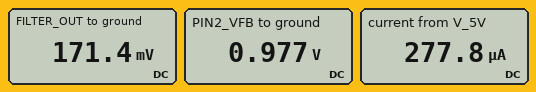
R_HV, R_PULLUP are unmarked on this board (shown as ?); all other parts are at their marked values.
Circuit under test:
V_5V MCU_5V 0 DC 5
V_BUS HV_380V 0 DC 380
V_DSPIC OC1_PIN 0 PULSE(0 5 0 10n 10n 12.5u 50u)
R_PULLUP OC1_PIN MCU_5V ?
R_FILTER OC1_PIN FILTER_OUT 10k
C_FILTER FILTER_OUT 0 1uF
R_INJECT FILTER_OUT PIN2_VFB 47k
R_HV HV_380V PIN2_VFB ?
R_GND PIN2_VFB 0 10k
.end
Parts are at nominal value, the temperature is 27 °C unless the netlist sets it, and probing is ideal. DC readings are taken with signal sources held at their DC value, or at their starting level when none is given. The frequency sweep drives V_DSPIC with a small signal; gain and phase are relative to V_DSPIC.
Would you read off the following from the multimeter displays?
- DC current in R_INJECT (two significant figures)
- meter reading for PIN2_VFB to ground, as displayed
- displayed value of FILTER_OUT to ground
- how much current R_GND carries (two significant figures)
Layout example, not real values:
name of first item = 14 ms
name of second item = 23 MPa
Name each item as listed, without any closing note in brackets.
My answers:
DC current in R_INJECT = 17 µA
meter reading for PIN2_VFB to ground, as displayed = 0.977 V
displayed value of FILTER_OUT to ground = 171.4 mV
how much current R_GND carries = 98 µA
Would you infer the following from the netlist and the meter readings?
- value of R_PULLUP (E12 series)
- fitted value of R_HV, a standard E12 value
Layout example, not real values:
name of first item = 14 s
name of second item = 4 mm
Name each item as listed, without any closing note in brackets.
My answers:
value of R_PULLUP = 18 kΩ
fitted value of R_HV, a standard E12 value = 3.3 MΩ
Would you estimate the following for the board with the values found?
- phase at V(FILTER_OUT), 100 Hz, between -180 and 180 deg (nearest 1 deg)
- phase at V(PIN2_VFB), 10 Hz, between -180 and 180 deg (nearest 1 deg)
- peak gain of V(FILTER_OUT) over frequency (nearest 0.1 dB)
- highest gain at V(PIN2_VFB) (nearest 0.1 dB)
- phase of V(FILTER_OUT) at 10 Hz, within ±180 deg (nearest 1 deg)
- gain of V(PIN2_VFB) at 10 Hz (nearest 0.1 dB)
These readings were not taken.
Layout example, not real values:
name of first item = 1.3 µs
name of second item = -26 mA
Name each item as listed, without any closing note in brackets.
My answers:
phase at V(FILTER_OUT), 100 Hz, between -180 and 180 deg = -79 deg
phase at V(PIN2_VFB), 10 Hz, between -180 and 180 deg = -28 deg
peak gain of V(FILTER_OUT) over frequency = -1.4 dB
highest gain at V(PIN2_VFB) = -16.5 dB
phase of V(FILTER_OUT) at 10 Hz, within ±180 deg = -28 deg
gain of V(PIN2_VFB) at 10 Hz = -17.6 dB
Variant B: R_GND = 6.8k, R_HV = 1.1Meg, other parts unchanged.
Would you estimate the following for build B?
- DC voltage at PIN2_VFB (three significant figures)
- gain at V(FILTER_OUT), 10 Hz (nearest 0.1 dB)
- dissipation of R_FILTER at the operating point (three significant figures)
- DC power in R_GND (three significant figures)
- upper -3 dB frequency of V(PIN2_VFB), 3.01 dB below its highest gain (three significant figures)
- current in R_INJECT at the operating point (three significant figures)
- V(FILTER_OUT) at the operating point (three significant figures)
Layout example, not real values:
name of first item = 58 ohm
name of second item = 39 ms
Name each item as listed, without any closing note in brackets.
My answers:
DC voltage at PIN2_VFB = 2.09 V
gain at V(FILTER_OUT), 10 Hz = -2.6 dB
dissipation of R_FILTER at the operating point = 13.4 µW
DC power in R_GND = 641 µW
upper -3 dB frequency of V(PIN2_VFB), 3.01 dB below its highest gain = 18.9 Hz
current in R_INJECT at the operating point = 36.6 µA
V(FILTER_OUT) at the operating point = 366 mV
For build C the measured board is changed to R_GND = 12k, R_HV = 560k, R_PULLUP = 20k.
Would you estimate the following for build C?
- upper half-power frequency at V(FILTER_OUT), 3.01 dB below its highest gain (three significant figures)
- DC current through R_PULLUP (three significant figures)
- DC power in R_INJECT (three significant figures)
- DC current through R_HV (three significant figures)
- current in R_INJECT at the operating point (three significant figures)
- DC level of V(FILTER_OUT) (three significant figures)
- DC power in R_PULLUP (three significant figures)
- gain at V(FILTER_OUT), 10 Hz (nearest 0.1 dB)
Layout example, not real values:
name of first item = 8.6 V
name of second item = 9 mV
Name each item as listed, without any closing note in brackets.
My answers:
upper half-power frequency at V(FILTER_OUT), 3.01 dB below its highest gain = 18.6 Hz
DC current through R_PULLUP = 250 µA
DC power in R_INJECT = 632 µW
DC current through R_HV = 667 µA
current in R_INJECT at the operating point = 116 µA
DC level of V(FILTER_OUT) = 1.16 V
DC power in R_PULLUP = 1.25 mW
gain at V(FILTER_OUT), 10 Hz = -2.5 dB
